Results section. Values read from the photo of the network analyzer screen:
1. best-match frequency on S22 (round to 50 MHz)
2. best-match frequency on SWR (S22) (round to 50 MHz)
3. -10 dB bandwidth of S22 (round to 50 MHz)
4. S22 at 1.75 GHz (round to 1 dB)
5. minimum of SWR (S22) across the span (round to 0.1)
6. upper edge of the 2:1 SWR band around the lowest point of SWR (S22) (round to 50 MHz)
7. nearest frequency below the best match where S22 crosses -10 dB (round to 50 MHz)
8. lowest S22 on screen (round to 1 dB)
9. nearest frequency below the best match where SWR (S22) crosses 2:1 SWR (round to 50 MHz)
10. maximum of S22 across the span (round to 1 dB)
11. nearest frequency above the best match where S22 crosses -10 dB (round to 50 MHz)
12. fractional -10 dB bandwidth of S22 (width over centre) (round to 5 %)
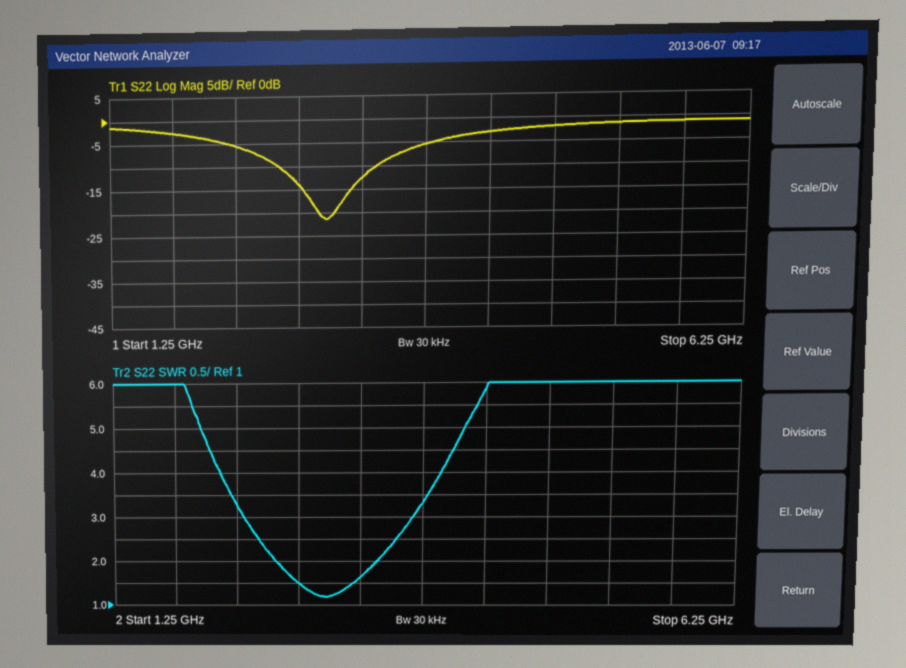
2.95 GHz
2.95 GHz
750 MHz
-3 dB
1.2
3.40 GHz
2.60 GHz
-21 dB
2.55 GHz
-1 dB
3.35 GHz
25 %
